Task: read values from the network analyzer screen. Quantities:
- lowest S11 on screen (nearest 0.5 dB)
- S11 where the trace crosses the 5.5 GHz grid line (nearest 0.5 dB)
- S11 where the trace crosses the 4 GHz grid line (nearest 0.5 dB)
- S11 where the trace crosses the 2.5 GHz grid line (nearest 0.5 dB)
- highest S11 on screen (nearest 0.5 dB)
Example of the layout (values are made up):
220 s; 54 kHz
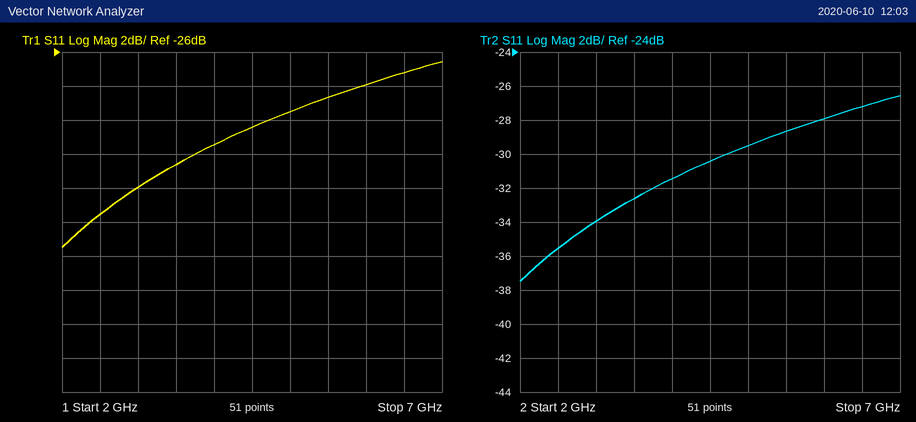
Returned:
-37.5 dB; -28.5 dB; -31.5 dB; -35.5 dB; -26.5 dB
